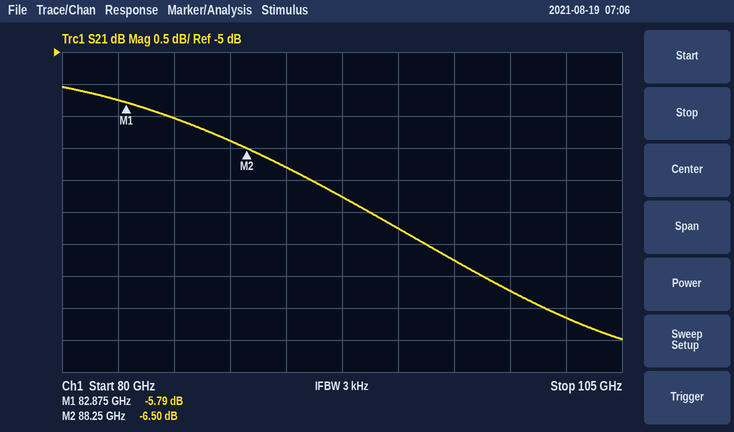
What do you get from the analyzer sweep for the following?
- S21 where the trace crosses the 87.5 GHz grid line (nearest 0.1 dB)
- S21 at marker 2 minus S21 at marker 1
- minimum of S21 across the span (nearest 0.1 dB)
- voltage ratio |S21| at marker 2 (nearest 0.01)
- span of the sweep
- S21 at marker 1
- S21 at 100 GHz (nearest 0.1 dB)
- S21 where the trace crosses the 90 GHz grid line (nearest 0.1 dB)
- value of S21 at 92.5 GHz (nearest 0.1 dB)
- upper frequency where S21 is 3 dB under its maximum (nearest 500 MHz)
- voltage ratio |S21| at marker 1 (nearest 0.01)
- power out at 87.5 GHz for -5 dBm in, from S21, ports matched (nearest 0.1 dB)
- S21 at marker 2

-6.4 dB
-0.71 dB
-9.5 dB
0.47
25 GHz
-5.79 dB
-8.7 dB
-6.8 dB
-7.3 dB
99.0 GHz
0.51
-11.4 dBm
-6.50 dB
